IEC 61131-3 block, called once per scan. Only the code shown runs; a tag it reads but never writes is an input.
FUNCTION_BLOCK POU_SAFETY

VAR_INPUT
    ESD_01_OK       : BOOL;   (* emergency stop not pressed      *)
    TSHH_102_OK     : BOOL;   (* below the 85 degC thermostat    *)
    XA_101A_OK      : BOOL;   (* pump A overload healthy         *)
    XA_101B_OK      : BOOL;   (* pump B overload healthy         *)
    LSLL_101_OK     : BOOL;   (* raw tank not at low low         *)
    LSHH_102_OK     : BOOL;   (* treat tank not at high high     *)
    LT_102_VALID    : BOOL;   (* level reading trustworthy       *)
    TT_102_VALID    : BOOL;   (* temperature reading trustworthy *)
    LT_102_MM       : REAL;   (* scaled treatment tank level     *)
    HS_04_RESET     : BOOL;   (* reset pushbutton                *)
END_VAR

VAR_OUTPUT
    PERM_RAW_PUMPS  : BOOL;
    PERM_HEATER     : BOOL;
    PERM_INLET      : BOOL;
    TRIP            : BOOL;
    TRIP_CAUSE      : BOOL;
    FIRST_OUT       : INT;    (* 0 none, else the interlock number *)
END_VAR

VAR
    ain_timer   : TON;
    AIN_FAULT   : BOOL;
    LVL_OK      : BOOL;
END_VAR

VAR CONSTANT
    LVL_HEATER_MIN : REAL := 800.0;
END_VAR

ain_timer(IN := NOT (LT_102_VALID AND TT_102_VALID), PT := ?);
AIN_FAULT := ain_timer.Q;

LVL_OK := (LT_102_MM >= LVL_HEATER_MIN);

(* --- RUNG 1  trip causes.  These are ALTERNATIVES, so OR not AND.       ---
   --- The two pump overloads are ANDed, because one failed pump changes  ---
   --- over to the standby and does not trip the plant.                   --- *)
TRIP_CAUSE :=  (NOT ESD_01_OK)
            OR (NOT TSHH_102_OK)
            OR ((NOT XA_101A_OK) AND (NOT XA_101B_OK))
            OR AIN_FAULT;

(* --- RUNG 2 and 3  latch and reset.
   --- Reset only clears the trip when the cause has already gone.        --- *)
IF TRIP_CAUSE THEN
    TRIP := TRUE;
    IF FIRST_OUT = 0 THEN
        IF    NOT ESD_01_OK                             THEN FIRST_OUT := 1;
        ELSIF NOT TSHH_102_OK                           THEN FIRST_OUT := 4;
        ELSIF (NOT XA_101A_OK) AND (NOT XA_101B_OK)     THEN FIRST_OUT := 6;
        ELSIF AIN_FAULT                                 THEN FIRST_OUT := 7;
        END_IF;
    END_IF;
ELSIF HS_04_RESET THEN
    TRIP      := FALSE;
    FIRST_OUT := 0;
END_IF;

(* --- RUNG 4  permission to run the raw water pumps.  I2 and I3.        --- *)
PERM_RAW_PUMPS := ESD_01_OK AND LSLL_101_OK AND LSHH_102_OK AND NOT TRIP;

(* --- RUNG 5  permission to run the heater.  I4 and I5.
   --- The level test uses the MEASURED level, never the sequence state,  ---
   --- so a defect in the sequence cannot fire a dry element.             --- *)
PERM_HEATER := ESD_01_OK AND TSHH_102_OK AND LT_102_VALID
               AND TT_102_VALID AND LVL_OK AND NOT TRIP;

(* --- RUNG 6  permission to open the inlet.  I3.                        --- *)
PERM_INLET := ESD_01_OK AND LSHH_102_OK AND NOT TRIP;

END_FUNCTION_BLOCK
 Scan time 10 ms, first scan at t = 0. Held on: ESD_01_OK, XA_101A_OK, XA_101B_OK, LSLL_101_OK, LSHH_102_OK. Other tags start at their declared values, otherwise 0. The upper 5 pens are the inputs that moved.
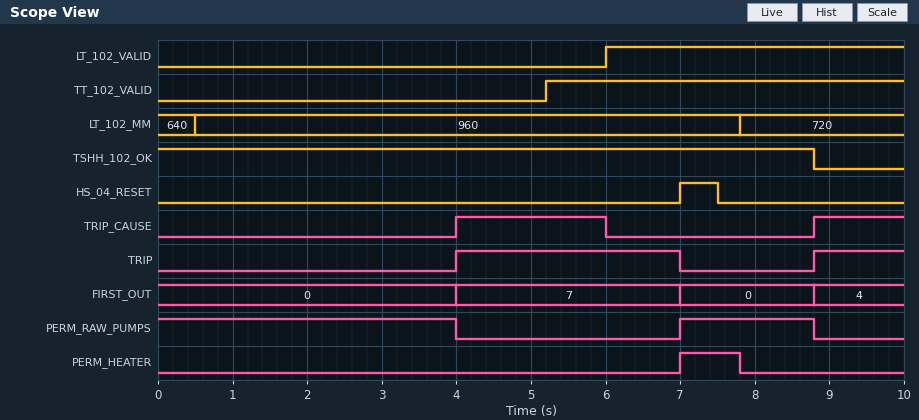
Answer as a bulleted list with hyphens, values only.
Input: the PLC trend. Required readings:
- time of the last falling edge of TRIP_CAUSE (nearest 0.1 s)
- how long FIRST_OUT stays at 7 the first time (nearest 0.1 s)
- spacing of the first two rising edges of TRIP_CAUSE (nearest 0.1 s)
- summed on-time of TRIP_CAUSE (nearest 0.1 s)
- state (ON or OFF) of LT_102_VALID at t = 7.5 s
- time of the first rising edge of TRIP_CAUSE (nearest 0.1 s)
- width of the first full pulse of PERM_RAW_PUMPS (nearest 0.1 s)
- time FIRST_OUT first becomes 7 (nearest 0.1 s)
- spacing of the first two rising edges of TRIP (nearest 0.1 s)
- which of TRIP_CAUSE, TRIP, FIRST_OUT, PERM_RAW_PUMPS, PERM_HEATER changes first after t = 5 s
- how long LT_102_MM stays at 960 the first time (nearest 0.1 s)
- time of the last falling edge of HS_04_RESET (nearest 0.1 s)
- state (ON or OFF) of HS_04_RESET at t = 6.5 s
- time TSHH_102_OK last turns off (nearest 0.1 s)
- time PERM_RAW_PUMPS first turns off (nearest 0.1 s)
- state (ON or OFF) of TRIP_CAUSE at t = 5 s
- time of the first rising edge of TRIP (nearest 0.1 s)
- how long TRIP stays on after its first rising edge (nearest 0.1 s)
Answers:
- 6.0 s
- 3.0 s
- 4.8 s
- 3.2 s
- ON
- 4.0 s
- 1.8 s
- 4.0 s
- 4.8 s
- TRIP_CAUSE
- 7.3 s
- 7.5 s
- OFF
- 8.8 s
- 4.0 s
- ON
- 4.0 s
- 3.0 s
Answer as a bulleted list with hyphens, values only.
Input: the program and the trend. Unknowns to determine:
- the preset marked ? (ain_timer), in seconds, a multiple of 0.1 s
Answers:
- 4.0 s
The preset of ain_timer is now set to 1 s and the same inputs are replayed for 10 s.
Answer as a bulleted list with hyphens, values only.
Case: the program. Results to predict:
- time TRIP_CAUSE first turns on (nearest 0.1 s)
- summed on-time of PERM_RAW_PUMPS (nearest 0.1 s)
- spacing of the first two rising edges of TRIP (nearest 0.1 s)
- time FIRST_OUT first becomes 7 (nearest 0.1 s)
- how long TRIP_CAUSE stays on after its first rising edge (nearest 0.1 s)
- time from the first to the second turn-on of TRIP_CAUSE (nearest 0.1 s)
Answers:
- 1.0 s
- 2.8 s
- 7.8 s
- 1.0 s
- 5.0 s
- 7.8 s
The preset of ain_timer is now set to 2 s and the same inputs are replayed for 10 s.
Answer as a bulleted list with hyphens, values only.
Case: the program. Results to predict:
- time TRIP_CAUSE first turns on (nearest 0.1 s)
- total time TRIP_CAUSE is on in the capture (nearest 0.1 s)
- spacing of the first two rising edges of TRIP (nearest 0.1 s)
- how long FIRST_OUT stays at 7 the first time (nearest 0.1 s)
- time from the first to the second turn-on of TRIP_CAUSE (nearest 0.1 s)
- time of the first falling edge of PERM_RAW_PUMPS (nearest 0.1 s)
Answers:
- 2.0 s
- 5.2 s
- 6.8 s
- 5.0 s
- 6.8 s
- 2.0 s
